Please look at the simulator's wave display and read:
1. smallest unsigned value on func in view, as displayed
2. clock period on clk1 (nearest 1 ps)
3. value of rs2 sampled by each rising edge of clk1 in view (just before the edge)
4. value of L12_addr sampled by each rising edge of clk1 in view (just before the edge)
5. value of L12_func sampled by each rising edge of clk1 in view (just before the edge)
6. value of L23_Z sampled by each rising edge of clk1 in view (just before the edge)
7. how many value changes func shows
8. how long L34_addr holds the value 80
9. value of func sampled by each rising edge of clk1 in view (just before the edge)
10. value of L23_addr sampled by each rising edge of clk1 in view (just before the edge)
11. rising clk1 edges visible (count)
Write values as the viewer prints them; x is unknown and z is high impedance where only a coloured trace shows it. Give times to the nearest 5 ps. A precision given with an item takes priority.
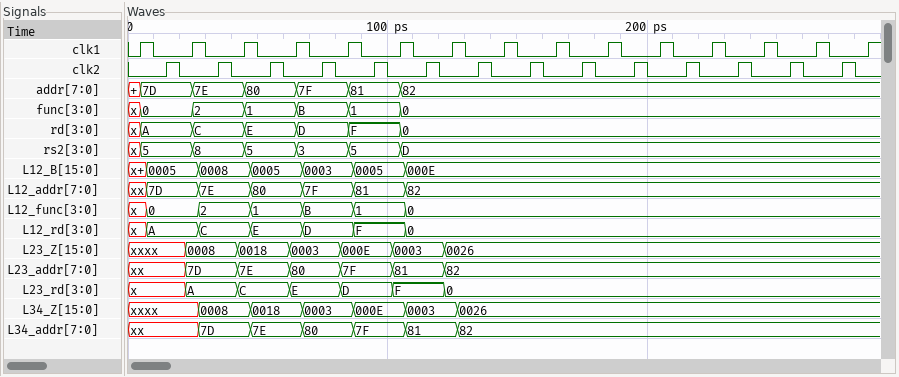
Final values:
0
20 ps
x, 5, 8, 5, 3, 5, D, D, D, D, D, D, D, D, D
xx, 7D, 7E, 80, 7F, 81, 82, 82, 82, 82, 82, 82, 82, 82, 82
x, 0, 2, 1, B, 1, 0, 0, 0, 0, 0, 0, 0, 0, 0
xxxx, 0008, 0018, 0003, 000E, 0003, 0026, 0026, 0026, 0026, 0026, 0026, 0026, 0026, 0026
6
20 ps
x, 0, 2, 1, B, 1, 0, 0, 0, 0, 0, 0, 0, 0, 0
xx, 7D, 7E, 80, 7F, 81, 82, 82, 82, 82, 82, 82, 82, 82, 82
15
